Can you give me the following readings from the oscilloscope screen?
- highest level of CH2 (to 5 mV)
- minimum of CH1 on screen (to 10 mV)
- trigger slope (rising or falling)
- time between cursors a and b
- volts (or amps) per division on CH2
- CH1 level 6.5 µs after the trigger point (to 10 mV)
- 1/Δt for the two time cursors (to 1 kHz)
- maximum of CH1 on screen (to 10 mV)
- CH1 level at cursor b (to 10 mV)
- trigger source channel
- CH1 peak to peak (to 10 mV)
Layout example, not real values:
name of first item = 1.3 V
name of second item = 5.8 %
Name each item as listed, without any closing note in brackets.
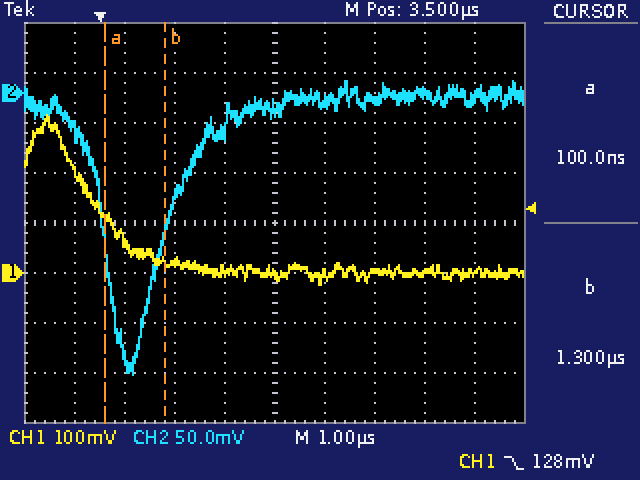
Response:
highest level of CH2 = 10 mV
minimum of CH1 on screen = -20 mV
trigger slope = falling
time between cursors a and b = 1.2 µs
volts (or amps) per division on CH2 = 50 mV
CH1 level 6.5 µs after the trigger point = 0 mV
1/Δt for the two time cursors = 833 kHz
maximum of CH1 on screen = 320 mV
CH1 level at cursor b = 20 mV
trigger source channel = CH1
CH1 peak to peak = 340 mV
